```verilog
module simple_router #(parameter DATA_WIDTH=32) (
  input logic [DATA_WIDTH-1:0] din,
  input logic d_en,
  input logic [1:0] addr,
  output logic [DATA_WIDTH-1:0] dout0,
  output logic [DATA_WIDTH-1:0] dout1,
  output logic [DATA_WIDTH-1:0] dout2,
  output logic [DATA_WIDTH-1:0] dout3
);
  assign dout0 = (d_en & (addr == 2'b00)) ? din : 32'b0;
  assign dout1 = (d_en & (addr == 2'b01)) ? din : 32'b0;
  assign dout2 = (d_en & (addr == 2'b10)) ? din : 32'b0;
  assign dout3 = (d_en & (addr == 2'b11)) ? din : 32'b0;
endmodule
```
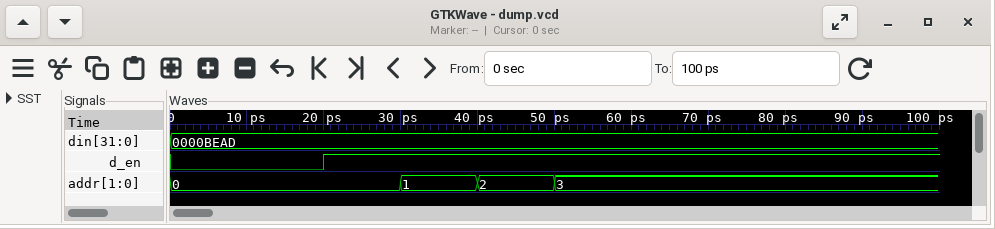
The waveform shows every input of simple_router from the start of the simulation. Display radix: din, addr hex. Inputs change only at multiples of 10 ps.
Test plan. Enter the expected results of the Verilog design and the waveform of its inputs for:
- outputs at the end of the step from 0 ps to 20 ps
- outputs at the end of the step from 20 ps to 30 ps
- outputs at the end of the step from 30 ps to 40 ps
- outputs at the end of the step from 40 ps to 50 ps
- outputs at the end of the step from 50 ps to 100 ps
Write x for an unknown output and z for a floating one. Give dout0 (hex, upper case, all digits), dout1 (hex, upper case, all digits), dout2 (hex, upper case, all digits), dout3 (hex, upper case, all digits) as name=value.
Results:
dout0=00000000, dout1=00000000, dout2=00000000, dout3=00000000
dout0=0000BEAD, dout1=00000000, dout2=00000000, dout3=00000000
dout0=00000000, dout1=0000BEAD, dout2=00000000, dout3=00000000
dout0=00000000, dout1=00000000, dout2=0000BEAD, dout3=00000000
dout0=00000000, dout1=00000000, dout2=00000000, dout3=0000BEAD
